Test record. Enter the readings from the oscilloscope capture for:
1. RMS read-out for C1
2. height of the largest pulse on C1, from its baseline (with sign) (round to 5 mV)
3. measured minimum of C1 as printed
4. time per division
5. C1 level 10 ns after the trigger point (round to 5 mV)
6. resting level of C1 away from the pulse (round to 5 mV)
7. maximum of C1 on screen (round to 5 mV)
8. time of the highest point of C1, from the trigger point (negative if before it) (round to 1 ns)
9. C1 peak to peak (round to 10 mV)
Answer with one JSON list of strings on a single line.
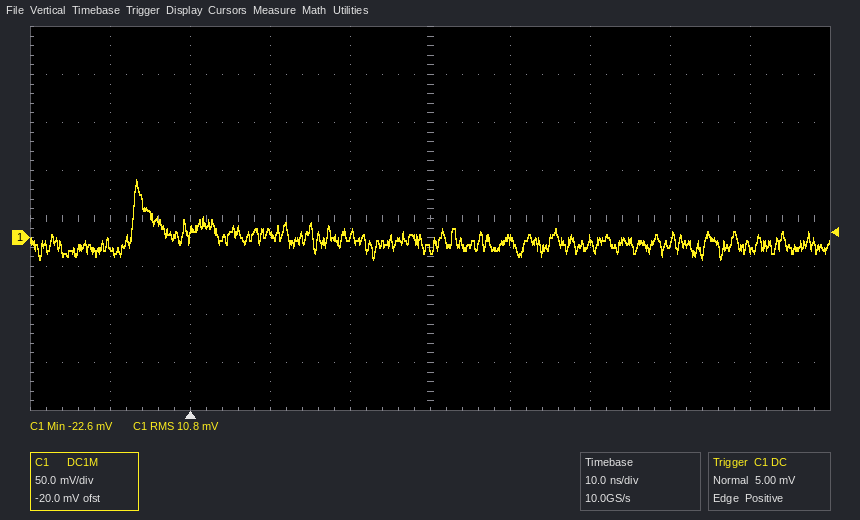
["10.8 mV", "+65 mV", "-22.6 mV", "10 ns", "5 mV", "-5 mV", "60 mV", "-7 ns", "80 mV"]
